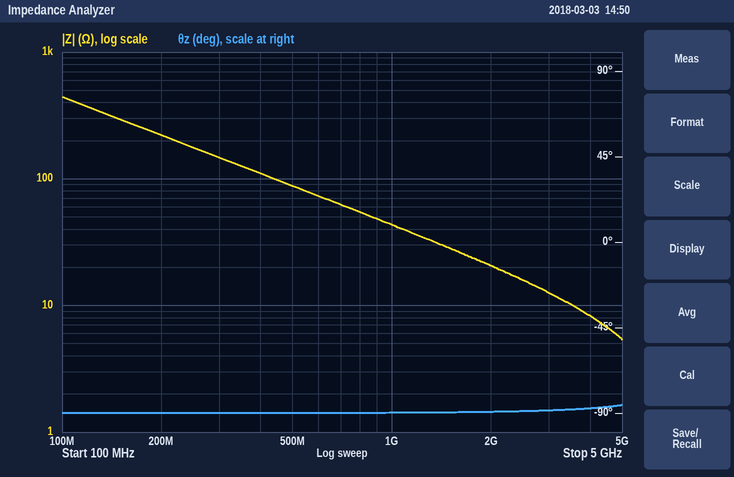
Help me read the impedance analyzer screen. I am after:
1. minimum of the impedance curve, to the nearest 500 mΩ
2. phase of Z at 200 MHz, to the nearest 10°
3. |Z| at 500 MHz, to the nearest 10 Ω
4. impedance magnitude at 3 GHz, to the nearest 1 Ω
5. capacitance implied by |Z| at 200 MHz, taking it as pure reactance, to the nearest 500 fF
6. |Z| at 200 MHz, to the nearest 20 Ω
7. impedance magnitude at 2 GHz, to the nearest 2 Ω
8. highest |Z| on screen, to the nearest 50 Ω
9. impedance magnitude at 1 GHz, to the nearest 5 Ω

5.5 Ω
-90°
90 Ω
13 Ω
3.5 pF
220 Ω
20 Ω
450 Ω
45 Ω
